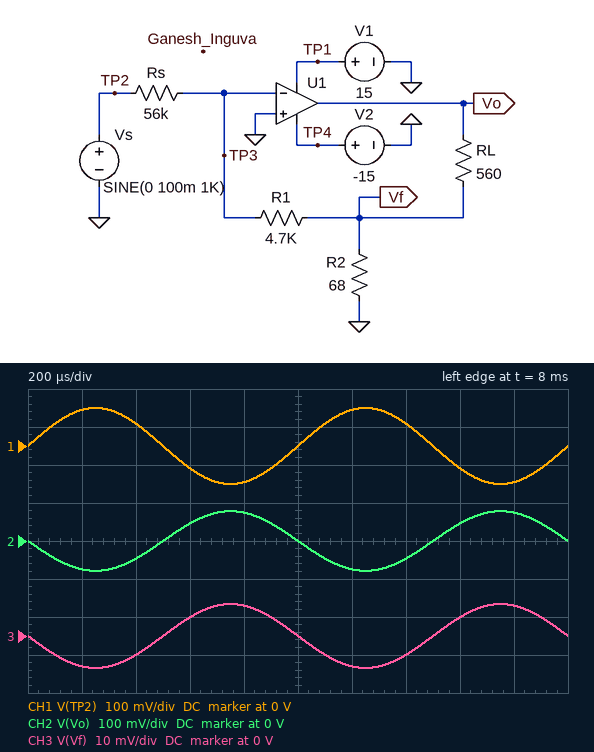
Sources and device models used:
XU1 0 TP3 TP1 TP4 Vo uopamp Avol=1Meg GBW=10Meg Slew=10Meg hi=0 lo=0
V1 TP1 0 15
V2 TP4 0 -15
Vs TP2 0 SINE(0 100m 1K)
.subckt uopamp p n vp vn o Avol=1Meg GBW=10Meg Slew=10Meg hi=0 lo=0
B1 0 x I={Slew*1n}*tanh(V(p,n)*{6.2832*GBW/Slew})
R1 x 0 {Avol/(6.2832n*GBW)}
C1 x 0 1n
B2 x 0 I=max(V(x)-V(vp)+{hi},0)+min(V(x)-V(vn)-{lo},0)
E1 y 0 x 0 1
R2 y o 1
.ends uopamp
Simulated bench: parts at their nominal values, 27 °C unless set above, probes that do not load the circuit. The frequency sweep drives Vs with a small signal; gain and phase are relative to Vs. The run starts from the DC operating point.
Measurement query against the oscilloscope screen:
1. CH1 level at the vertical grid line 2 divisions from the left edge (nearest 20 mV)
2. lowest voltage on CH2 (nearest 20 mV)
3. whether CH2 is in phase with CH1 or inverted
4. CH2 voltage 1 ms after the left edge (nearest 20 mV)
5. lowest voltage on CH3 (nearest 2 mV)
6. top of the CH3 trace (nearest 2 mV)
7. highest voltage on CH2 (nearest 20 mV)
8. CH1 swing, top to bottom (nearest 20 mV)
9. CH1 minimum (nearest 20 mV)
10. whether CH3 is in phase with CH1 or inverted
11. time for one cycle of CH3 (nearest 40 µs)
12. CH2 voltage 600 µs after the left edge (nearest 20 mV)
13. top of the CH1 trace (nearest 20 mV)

60 mV
-80 mV
inverted
0 V
-8 mV
8 mV
80 mV
200 mV
-100 mV
inverted
1.00 ms
40 mV
100 mV
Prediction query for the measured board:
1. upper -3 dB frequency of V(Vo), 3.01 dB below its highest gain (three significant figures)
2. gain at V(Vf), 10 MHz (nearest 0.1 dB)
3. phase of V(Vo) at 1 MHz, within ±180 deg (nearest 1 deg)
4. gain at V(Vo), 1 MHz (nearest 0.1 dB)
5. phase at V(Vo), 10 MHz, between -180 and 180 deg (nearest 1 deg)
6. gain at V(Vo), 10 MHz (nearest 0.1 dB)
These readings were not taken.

996 kHz
-41.5 dB
135 deg
-5.1 dB
96 deg
-22.2 dB
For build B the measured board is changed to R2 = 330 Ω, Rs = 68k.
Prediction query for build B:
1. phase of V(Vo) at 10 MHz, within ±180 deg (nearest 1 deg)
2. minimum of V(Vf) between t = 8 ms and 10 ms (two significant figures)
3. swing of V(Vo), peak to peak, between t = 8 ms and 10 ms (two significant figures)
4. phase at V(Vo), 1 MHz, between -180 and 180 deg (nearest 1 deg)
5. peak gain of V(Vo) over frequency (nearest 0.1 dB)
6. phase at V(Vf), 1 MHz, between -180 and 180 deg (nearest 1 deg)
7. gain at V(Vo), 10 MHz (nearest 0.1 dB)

109 deg
-6.9 mV
39 mV
164 deg
-14.2 dB
163 deg
-23.9 dB
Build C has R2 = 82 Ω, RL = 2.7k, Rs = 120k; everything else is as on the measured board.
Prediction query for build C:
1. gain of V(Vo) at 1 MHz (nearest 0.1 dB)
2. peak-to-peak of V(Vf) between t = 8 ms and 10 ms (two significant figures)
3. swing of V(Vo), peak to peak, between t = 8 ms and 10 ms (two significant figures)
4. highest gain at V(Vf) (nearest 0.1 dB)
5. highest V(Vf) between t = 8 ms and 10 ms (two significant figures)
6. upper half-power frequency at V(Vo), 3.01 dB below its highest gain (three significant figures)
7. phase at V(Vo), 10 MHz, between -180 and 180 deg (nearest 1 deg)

-8.7 dB
7.8 mV
270 mV
-28.1 dB
3.9 mV
283 kHz
92 deg
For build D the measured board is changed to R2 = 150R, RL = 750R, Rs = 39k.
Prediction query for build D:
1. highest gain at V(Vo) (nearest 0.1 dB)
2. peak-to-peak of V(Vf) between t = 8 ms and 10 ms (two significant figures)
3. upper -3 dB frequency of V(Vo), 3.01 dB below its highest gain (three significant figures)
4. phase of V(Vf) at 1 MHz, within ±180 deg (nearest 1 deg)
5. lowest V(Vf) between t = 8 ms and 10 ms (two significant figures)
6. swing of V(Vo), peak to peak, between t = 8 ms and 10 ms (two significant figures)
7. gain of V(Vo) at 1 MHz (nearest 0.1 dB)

-2.6 dB
24 mV
1.48 MHz
145 deg
-12 mV
150 mV
-4.2 dB
